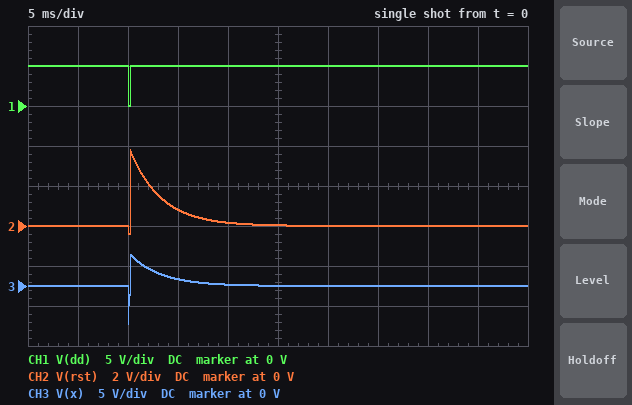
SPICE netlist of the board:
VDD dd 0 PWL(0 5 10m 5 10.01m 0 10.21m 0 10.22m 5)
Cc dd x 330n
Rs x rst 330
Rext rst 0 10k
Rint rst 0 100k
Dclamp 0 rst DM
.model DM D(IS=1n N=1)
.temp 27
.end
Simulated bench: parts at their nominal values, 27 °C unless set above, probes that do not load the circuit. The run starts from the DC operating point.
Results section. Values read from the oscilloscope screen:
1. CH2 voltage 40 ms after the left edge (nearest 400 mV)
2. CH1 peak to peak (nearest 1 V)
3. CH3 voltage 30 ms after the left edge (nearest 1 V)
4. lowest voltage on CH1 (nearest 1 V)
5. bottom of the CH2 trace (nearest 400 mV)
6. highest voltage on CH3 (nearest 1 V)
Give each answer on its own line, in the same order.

0 V
5 V
0 V
0 V
-400 mV
4 V
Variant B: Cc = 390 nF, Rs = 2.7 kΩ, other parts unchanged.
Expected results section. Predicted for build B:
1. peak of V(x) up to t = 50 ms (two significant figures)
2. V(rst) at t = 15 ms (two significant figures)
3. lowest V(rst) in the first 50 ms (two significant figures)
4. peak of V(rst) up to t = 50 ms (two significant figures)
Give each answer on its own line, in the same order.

830 mV
230 mV
-370 mV
640 mV
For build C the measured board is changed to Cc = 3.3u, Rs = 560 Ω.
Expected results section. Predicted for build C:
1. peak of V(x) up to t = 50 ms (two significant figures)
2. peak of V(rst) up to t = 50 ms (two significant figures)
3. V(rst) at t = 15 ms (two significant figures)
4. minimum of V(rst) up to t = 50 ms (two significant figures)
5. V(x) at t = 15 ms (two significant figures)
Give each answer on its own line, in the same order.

490 mV
460 mV
400 mV
-410 mV
420 mV
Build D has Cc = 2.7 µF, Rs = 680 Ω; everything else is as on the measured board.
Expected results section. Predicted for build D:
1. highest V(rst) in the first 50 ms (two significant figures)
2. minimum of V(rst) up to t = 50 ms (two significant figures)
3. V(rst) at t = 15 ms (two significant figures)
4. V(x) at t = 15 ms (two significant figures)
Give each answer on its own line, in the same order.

460 mV
-410 mV
380 mV
410 mV
